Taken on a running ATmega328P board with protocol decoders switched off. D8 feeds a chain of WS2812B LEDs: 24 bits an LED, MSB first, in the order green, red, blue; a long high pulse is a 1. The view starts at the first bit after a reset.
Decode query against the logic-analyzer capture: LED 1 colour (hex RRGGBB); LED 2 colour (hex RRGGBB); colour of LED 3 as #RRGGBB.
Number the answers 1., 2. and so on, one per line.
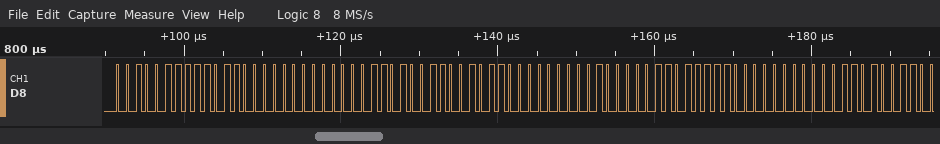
1. #D82700
2. #CB3400
3. #BE4100
